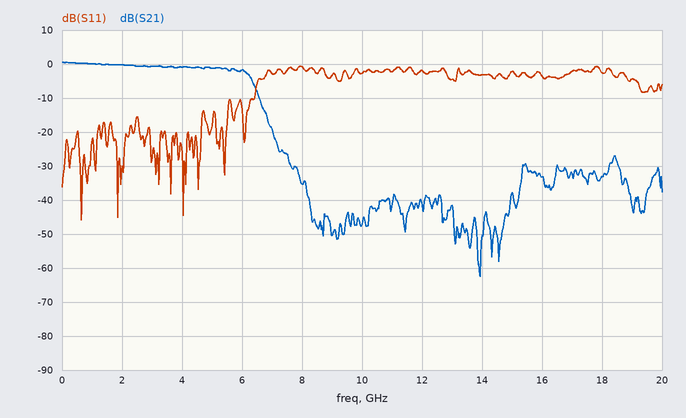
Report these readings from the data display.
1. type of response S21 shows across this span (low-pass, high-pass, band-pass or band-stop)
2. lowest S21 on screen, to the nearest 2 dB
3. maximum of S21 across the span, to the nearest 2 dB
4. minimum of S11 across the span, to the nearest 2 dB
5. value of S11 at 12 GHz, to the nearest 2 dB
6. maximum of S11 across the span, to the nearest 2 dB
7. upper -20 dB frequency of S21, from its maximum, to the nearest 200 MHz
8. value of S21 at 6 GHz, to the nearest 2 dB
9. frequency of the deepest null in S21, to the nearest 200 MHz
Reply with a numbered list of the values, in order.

1. low-pass
2. -62 dB
3. 0 dB
4. -46 dB
5. -2 dB
6. 0 dB
7. 7.0 GHz
8. -2 dB
9. 14.0 GHz
